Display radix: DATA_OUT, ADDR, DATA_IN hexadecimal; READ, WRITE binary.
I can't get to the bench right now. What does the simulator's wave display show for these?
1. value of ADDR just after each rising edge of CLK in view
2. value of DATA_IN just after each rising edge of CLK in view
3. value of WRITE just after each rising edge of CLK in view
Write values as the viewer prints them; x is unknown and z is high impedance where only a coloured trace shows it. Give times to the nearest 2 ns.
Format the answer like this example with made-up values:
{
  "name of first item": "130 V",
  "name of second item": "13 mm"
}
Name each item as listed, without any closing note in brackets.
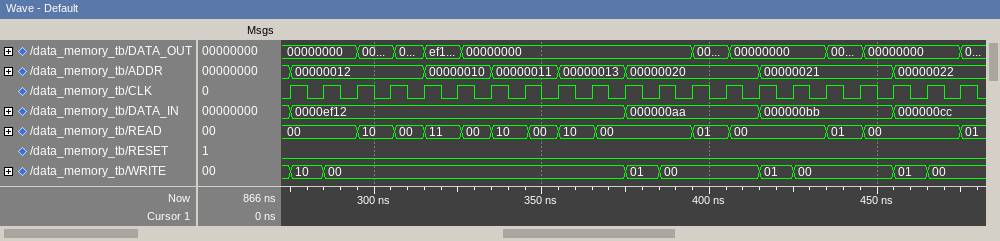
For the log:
{
  "value of ADDR just after each rising edge of CLK in view": "00000012, 00000012, 00000012, 00000012, 00000010, 00000010, 00000011, 00000011, 00000013, 00000013, 00000020, 00000020, 00000020, 00000020, 00000021, 00000021, 00000021, 00000021, 00000022, 00000022, 00000022",
  "value of DATA_IN just after each rising edge of CLK in view": "0000ef12, 0000ef12, 0000ef12, 0000ef12, 0000ef12, 0000ef12, 0000ef12, 0000ef12, 0000ef12, 0000ef12, 000000aa, 000000aa, 000000aa, 000000aa, 000000bb, 000000bb, 000000bb, 000000bb, 000000cc, 000000cc, 000000cc",
  "value of WRITE just after each rising edge of CLK in view": "10, 00, 00, 00, 00, 00, 00, 00, 00, 00, 01, 00, 00, 00, 01, 00, 00, 00, 01, 00, 00"
}
